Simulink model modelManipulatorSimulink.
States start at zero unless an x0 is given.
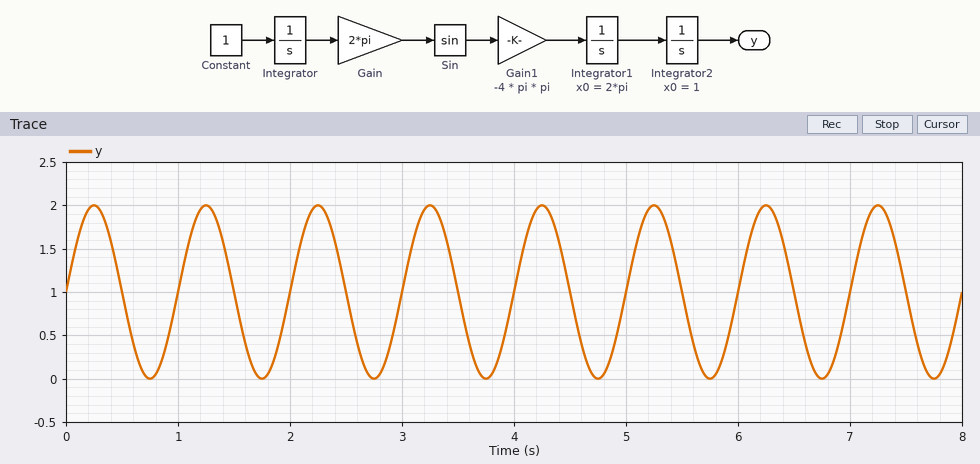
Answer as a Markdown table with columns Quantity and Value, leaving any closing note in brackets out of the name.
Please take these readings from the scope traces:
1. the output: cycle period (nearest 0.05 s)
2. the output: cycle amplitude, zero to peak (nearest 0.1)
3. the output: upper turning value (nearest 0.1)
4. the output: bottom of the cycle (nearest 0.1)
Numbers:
| Quantity | Value |
|---|---|
| the output: cycle period | 1.00 s |
| the output: cycle amplitude, zero to peak | 1.0 |
| the output: upper turning value | 2.0 |
| the output: bottom of the cycle | 0.0 |
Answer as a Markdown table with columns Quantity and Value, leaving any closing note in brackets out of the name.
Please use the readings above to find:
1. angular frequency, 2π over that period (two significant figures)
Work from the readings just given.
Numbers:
| Quantity | Value |
|---|---|
| angular frequency, 2π over that period | 6.3 rad/s |
